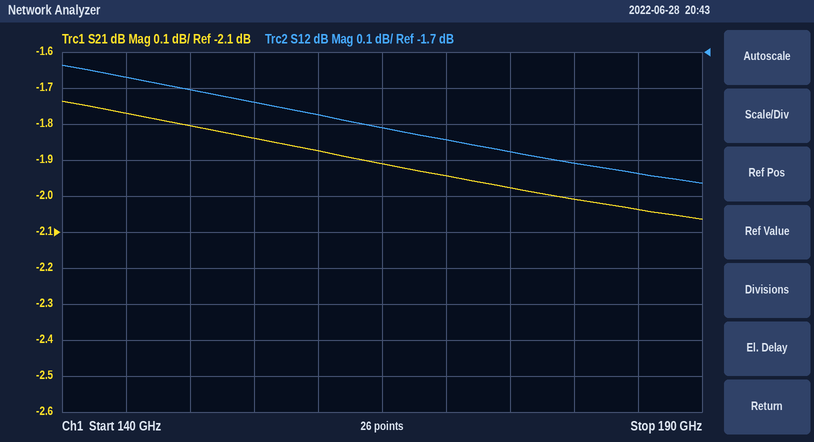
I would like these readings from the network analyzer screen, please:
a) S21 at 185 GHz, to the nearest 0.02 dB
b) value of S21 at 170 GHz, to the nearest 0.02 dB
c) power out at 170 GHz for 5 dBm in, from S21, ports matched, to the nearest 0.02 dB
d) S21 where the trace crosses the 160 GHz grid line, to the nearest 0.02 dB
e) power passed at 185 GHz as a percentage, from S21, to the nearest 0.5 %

-2.04 dB
-1.94 dB
3.06 dBm
-1.88 dB
62.5 %
